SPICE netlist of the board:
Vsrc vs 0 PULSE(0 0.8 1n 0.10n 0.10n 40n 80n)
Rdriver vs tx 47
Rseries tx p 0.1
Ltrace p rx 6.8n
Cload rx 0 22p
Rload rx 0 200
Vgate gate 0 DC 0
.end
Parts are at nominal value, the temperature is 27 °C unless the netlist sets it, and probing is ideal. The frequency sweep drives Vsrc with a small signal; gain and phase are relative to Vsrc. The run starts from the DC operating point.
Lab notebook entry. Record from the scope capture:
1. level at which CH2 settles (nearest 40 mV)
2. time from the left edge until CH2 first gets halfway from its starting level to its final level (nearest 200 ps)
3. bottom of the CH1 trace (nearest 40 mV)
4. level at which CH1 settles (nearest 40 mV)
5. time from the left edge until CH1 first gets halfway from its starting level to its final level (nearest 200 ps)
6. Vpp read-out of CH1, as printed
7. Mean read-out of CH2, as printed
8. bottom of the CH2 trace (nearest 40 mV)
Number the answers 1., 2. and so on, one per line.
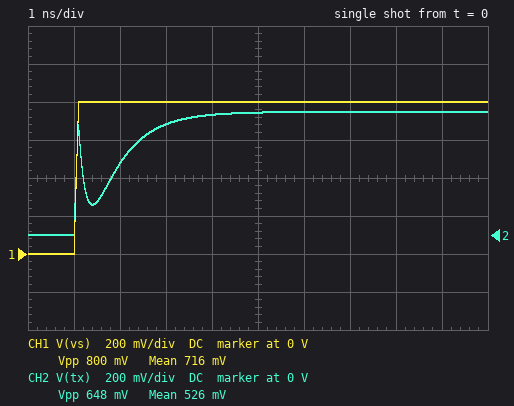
1. 640 mV
2. 1.0 ns
3. 0 V
4. 800 mV
5. 1.0 ns
6. 800 mV
7. 526 mV
8. 0 V
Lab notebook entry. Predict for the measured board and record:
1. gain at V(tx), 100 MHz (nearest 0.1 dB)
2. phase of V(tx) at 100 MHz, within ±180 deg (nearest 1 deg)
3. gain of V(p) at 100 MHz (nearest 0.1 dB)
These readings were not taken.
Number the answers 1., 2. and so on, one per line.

1. -3.2 dB
2. -28 deg
3. -3.2 dB
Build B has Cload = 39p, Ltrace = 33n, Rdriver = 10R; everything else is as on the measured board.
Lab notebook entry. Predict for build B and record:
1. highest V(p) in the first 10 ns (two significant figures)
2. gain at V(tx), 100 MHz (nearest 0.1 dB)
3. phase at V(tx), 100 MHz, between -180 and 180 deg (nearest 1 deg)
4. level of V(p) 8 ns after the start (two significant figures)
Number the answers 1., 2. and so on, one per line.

1. 850 mV
2. -2.2 dB
3. -21 deg
4. 780 mV
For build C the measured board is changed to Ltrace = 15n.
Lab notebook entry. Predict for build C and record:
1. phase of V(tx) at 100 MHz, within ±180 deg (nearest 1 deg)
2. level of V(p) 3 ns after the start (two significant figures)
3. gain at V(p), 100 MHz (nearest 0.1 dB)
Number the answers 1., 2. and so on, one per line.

1. -29 deg
2. 560 mV
3. -3.5 dB
